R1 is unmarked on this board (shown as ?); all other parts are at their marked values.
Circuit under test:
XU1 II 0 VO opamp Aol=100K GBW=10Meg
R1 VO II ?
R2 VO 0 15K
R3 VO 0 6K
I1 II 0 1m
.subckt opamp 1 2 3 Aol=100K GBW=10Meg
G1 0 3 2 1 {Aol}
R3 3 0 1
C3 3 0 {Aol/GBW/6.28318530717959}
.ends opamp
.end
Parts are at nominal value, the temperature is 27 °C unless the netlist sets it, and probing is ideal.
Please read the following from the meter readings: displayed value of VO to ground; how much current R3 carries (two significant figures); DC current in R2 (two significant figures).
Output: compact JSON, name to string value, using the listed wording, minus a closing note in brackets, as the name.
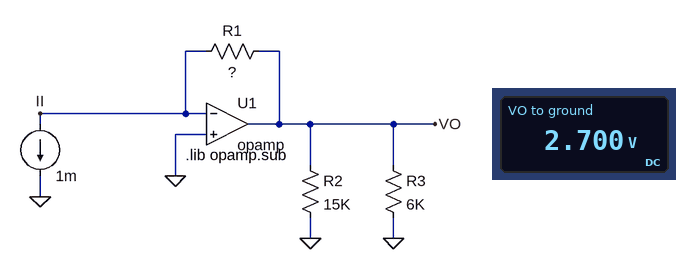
{"displayed value of VO to ground": "2.700 V", "how much current R3 carries": "450 µA", "DC current in R2": "180 µA"}
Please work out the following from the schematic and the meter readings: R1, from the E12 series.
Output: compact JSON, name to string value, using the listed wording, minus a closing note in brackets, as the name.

{"R1, from the E12 series": "2.7 kΩ"}
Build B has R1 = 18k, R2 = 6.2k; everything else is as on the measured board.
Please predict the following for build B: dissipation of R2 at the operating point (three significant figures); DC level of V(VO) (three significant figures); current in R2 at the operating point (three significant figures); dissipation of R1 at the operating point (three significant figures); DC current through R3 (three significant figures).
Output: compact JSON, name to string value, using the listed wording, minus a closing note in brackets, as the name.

{"dissipation of R2 at the operating point": "52.3 mW", "DC level of V(VO)": "18.0 V", "current in R2 at the operating point": "2.90 mA", "dissipation of R1 at the operating point": "18.0 mW", "DC current through R3": "3.00 mA"}
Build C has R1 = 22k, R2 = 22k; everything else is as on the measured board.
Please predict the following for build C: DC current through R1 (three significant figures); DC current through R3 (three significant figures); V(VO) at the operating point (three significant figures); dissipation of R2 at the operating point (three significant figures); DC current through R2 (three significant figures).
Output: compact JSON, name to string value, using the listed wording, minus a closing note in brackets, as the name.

{"DC current through R1": "1.00 mA", "DC current through R3": "3.67 mA", "V(VO) at the operating point": "22.0 V", "dissipation of R2 at the operating point": "22.0 mW", "DC current through R2": "1.00 mA"}
